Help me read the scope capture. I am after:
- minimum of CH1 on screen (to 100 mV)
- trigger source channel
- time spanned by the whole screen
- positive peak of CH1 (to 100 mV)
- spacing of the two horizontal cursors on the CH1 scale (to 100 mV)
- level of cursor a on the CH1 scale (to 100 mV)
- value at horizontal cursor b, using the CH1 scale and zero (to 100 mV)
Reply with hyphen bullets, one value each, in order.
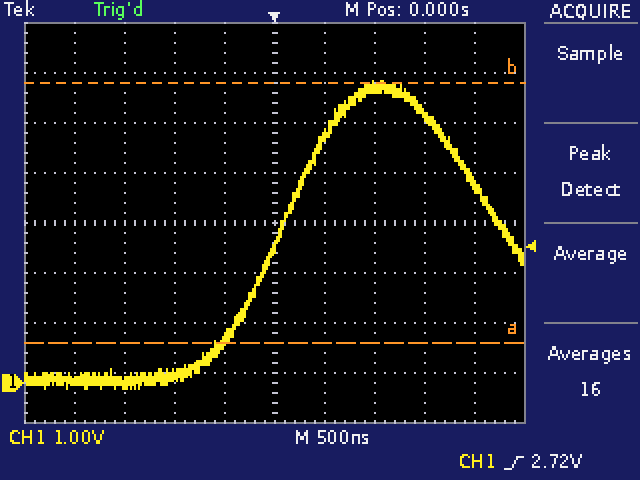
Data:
- -100 mV
- CH1
- 5 µs
- 6.0 V
- 5.2 V
- 800 mV
- 6.0 V
